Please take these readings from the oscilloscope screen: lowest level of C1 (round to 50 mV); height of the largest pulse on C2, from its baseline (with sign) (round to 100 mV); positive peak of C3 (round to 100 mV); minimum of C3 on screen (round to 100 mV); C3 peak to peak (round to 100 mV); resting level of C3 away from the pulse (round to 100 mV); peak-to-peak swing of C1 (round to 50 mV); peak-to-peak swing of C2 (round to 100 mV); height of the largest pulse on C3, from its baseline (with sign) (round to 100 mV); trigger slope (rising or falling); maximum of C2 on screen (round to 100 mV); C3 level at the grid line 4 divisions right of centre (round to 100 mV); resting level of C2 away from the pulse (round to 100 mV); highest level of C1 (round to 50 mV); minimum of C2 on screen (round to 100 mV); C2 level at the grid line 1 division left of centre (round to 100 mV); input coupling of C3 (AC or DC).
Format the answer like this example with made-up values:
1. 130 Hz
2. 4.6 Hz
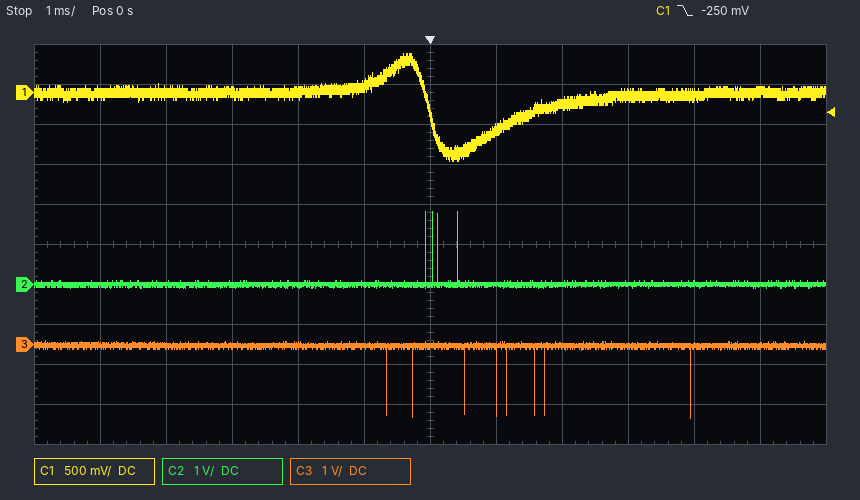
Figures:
1. -850 mV
2. +1.8 V
3. 100 mV
4. -1.8 V
5. 1.9 V
6. 0.0 V
7. 1.35 V
8. 1.9 V
9. -1.8 V
10. falling
11. 1.8 V
12. 0.0 V
13. 0.0 V
14. 500 mV
15. -100 mV
16. 0.0 V
17. DC
